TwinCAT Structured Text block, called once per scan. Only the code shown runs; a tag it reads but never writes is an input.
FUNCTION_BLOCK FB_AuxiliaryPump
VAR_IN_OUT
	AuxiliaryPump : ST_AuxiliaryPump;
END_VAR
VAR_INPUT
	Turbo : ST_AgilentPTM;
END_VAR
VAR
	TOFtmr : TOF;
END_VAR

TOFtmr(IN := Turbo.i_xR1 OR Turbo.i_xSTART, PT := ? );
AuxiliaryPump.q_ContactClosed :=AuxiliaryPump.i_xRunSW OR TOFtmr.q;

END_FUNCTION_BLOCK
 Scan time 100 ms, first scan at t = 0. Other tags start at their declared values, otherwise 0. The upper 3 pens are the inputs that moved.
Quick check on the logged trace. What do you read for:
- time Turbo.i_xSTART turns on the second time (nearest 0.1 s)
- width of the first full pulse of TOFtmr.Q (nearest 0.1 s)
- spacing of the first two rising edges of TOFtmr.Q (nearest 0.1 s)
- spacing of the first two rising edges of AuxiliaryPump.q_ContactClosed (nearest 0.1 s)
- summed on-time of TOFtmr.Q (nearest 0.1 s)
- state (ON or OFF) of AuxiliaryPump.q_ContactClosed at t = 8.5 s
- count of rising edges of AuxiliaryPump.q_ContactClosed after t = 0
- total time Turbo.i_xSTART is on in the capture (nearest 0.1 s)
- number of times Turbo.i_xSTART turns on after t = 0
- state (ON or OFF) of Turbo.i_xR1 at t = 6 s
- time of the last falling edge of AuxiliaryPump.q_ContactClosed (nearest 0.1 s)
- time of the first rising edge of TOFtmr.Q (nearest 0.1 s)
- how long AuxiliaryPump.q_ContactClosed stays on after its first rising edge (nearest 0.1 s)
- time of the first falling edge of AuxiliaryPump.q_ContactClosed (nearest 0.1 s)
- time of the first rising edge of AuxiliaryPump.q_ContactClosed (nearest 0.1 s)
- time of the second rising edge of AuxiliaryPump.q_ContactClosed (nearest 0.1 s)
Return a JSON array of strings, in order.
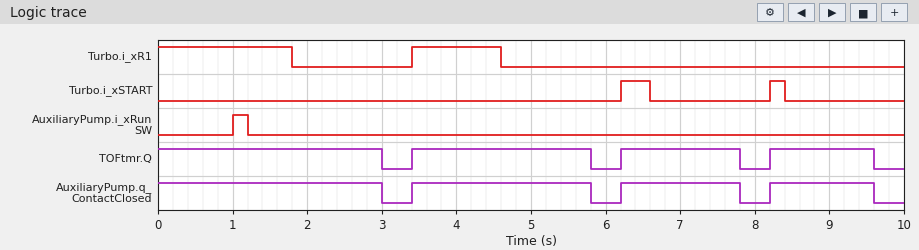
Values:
["8.2 s", "2.4 s", "2.8 s", "2.8 s", "8.4 s", "ON", "3", "0.6 s", "2", "OFF", "9.6 s", "3.4 s", "2.4 s", "3.0 s", "3.4 s", "6.2 s"]
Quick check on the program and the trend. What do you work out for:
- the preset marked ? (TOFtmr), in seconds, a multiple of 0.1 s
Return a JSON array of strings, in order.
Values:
["1.2 s"]
